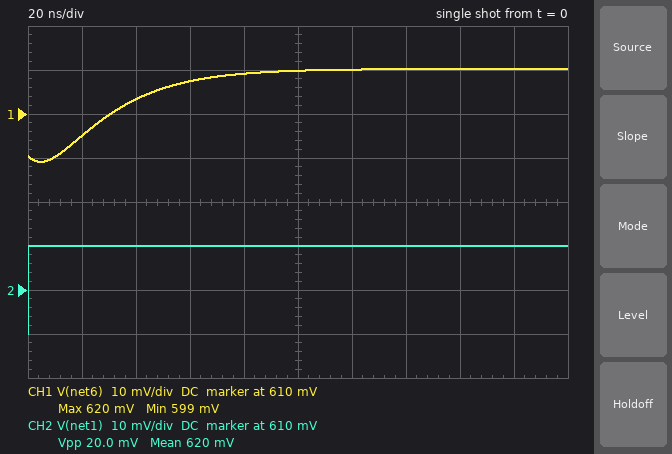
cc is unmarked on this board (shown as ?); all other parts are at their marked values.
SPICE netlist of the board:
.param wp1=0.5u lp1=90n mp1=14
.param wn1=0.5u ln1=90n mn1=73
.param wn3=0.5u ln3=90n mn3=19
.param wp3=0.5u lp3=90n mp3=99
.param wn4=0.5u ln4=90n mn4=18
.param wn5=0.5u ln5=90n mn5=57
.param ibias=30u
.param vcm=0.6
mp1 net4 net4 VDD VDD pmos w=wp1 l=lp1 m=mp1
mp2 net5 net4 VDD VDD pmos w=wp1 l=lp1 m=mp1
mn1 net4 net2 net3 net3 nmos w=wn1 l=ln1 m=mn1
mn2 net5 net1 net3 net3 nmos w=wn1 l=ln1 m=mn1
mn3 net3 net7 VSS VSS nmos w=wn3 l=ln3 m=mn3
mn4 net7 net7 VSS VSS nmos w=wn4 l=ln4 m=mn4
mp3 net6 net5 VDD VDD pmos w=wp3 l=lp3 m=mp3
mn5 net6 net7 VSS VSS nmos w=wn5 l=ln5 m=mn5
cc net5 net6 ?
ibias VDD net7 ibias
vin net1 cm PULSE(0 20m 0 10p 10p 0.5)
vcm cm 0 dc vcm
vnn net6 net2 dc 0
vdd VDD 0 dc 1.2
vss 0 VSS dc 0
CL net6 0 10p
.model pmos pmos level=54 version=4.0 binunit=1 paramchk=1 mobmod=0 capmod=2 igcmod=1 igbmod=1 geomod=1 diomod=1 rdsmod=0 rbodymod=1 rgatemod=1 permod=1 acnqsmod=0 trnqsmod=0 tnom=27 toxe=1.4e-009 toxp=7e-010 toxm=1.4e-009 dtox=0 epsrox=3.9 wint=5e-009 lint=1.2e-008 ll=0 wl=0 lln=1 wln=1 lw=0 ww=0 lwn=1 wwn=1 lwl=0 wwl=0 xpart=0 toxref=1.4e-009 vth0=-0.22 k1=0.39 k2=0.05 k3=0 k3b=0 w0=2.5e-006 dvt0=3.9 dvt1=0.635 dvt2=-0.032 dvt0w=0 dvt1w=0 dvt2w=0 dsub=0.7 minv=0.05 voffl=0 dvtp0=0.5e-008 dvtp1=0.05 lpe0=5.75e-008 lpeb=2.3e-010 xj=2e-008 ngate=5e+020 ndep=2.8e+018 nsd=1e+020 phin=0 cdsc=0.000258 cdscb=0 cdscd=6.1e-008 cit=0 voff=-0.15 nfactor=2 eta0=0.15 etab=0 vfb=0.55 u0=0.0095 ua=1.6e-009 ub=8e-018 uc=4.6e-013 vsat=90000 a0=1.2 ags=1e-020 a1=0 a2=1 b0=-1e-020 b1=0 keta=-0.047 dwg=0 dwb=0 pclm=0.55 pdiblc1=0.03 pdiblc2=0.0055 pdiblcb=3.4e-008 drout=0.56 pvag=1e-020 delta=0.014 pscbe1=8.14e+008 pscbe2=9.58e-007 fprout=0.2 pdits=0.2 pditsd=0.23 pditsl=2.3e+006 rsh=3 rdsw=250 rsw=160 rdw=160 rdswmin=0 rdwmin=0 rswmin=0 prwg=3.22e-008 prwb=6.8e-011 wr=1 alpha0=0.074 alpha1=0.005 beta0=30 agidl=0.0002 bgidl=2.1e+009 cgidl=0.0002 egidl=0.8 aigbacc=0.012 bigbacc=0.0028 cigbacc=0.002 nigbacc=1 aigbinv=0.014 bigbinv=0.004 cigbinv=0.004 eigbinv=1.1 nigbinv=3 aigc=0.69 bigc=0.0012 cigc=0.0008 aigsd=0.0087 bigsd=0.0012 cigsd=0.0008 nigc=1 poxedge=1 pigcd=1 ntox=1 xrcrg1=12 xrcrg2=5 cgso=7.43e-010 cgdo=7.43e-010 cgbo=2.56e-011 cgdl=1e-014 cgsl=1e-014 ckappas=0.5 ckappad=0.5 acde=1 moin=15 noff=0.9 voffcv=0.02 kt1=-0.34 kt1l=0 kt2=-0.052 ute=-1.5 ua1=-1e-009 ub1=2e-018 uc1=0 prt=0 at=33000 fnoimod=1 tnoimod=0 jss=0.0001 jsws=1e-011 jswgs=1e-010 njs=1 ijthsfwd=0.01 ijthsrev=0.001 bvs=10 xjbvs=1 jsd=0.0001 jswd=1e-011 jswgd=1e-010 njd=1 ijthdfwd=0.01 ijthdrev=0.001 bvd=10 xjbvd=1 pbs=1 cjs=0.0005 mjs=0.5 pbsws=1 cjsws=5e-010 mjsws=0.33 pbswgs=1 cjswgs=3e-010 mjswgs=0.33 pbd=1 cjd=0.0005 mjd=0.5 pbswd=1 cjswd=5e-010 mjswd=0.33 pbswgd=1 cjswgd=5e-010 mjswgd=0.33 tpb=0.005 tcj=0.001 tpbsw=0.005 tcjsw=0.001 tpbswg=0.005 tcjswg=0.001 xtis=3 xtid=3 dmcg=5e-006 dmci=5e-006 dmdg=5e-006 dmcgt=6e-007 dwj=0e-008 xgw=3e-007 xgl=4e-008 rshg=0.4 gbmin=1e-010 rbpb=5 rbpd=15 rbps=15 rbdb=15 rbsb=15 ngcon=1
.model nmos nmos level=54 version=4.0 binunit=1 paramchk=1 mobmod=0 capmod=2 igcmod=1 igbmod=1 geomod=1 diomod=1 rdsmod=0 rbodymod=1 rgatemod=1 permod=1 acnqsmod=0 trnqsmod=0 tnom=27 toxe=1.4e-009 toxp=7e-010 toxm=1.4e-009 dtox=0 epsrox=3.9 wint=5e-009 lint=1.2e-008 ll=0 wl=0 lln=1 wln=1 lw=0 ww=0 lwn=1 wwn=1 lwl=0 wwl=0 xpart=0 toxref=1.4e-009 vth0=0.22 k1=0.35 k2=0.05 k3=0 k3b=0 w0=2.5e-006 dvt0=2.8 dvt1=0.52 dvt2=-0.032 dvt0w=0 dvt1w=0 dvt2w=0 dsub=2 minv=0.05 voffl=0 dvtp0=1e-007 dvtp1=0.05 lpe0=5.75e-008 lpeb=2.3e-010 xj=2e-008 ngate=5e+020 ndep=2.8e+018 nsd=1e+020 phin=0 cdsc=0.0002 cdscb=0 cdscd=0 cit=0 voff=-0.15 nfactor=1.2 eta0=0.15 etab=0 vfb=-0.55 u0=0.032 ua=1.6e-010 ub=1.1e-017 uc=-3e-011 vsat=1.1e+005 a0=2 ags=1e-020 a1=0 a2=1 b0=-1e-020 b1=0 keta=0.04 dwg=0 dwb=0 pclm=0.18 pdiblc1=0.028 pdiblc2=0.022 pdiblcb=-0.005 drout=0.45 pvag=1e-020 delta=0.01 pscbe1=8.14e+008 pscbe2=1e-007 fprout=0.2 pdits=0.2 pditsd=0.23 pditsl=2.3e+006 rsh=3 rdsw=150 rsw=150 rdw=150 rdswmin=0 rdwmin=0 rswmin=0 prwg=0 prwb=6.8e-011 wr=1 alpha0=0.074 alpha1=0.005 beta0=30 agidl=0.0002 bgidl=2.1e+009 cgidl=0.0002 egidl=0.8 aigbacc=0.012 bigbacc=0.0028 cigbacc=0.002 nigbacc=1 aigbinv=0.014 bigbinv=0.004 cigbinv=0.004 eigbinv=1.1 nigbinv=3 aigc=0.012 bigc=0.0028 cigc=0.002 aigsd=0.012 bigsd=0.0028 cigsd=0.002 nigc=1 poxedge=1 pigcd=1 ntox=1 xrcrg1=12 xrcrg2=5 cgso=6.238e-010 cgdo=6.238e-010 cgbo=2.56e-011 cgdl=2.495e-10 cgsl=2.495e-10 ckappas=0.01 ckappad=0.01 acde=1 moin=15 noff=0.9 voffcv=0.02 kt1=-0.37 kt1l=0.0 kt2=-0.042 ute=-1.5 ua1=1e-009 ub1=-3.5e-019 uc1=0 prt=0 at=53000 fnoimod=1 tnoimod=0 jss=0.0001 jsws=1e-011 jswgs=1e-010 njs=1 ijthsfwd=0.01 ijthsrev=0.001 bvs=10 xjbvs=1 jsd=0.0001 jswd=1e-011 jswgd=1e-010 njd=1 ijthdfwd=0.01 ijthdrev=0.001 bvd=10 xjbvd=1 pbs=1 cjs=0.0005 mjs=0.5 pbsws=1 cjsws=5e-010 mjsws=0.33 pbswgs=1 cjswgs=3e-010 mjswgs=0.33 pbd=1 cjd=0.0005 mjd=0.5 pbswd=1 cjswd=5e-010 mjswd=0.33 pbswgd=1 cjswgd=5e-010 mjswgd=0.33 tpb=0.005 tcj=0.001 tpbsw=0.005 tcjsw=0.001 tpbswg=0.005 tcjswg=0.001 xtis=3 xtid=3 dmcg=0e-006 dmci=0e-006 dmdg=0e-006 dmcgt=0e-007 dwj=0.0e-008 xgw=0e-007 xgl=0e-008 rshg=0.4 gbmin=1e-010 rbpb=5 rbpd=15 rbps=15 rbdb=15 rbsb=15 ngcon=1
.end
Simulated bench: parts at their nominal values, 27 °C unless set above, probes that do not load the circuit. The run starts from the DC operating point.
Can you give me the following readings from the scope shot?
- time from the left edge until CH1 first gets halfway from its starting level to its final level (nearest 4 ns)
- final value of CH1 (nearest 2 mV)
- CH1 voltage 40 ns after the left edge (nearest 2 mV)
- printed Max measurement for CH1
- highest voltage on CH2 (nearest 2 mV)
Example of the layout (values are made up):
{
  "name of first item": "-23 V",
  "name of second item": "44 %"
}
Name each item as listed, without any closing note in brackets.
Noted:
{
  "time from the left edge until CH1 first gets halfway from its starting level to its final level": "32 ns",
  "final value of CH1": "620 mV",
  "CH1 voltage 40 ns after the left edge": "614 mV",
  "printed Max measurement for CH1": "620 mV",
  "highest voltage on CH2": "620 mV"
}
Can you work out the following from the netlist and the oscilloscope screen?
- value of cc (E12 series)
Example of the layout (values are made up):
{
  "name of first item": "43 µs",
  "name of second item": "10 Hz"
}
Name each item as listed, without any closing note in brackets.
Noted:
{
  "value of cc": "12 pF"
}
